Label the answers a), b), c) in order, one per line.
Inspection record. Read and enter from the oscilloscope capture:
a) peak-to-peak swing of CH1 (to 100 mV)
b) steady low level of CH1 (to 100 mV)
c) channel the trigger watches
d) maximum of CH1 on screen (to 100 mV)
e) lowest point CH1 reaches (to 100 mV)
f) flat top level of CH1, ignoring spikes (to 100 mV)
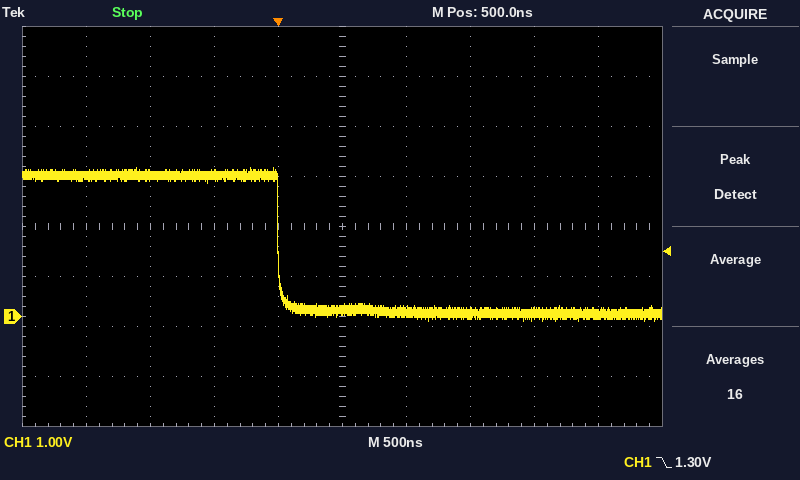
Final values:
a) 3.1 V
b) 100 mV
c) CH1
d) 3.0 V
e) -100 mV
f) 2.8 V
